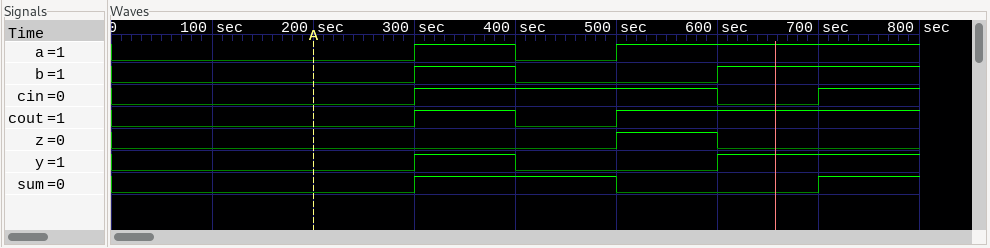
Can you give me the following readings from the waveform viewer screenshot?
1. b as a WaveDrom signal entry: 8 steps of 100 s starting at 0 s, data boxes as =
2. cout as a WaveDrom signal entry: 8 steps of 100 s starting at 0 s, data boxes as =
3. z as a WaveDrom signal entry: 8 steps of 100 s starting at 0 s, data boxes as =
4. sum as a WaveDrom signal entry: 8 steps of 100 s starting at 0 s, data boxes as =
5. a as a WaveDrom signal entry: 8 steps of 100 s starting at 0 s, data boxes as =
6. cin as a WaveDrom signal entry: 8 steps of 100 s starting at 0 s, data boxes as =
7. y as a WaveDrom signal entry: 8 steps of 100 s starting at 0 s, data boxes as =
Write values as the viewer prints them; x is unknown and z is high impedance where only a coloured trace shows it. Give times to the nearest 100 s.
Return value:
{name: 'b', wave: '0..10.1.'}
{name: 'cout', wave: '0..101..'}
{name: 'z', wave: '0....10.'}
{name: 'sum', wave: '0..1.0.1'}
{name: 'a', wave: '0..101..'}
{name: 'cin', wave: '0..1..01'}
{name: 'y', wave: '0..10.1.'}
